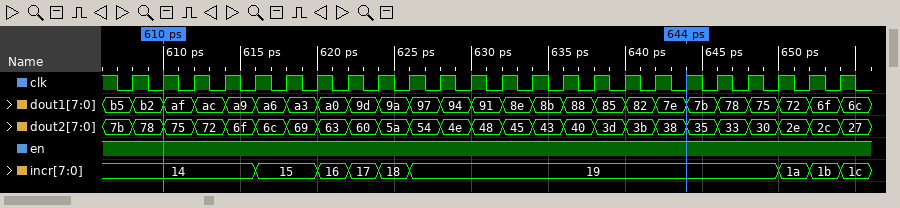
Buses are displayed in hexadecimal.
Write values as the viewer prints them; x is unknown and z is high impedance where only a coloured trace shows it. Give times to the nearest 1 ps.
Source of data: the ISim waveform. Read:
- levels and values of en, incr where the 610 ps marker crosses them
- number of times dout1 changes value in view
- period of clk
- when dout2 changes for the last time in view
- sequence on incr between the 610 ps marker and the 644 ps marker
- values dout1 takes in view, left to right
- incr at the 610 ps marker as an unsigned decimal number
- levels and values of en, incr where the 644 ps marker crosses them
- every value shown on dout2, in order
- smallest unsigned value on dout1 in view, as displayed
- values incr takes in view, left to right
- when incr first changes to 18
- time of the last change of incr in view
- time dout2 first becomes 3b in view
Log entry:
en=1, incr=14
24
2 ps
654 ps
14, 15, 16, 17, 18, 19
b5, b2, af, ac, a9, a6, a3, a0, 9d, 9a, 97, 94, 91, 8e, 8b, 88, 85, 82, 7e, 7b, 78, 75, 72, 6f, 6c
20
en=1, incr=19
7b, 78, 75, 72, 6f, 6c, 69, 63, 60, 5a, 54, 4e, 48, 45, 43, 40, 3d, 3b, 38, 35, 33, 30, 2e, 2c, 27
6c
14, 15, 16, 17, 18, 19, 1a, 1b, 1c
624 ps
654 ps
640 ps
